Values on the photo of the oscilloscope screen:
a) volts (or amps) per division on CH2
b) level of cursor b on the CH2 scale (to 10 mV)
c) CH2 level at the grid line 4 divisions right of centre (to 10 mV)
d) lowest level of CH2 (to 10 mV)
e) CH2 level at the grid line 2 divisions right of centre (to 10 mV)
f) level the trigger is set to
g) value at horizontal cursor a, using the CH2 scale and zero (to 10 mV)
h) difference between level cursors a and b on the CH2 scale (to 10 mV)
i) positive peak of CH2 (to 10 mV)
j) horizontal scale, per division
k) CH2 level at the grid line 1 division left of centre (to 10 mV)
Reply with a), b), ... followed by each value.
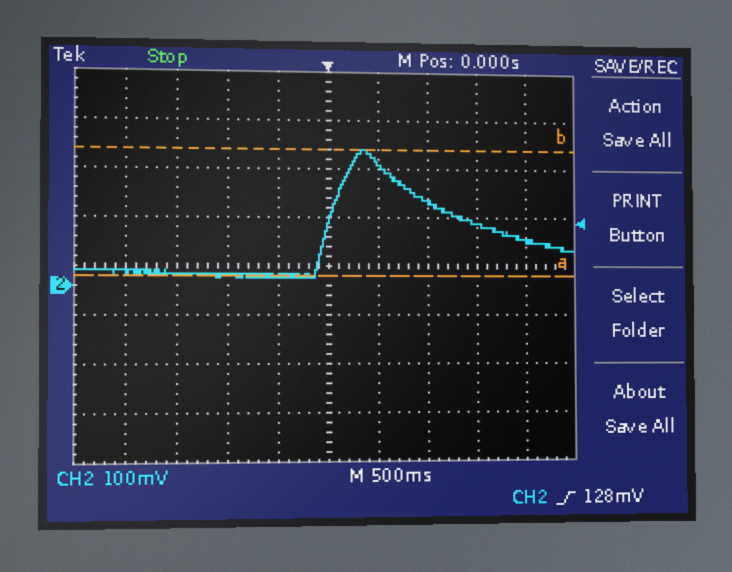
a) 100 mV
b) 280 mV
c) 90 mV
d) 20 mV
e) 170 mV
f) 128 mV
g) 20 mV
h) 260 mV
i) 280 mV
j) 500 ms
k) 20 mV
